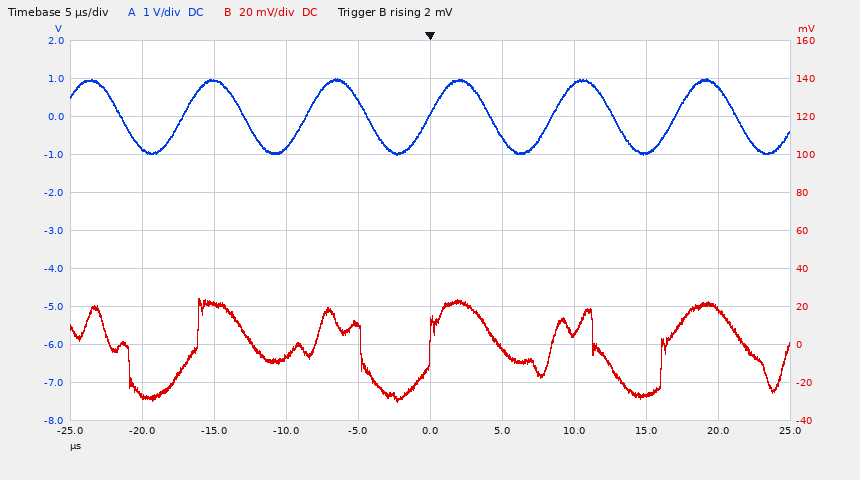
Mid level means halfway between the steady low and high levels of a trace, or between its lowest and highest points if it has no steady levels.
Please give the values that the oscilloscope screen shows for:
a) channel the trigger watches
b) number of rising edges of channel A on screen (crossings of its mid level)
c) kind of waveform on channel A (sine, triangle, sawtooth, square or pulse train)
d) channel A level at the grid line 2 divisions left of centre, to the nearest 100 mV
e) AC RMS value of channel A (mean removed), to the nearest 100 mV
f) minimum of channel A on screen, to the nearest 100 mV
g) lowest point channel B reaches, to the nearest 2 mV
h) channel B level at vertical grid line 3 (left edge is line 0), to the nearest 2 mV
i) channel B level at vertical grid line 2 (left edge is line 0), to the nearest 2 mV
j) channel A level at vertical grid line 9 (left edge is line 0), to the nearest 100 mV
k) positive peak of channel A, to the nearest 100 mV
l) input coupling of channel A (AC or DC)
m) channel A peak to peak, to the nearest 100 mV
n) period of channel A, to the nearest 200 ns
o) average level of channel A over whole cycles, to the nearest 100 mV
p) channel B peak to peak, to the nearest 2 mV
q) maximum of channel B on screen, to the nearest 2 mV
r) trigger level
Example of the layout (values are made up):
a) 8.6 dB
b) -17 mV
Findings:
a) channel B
b) 5
c) sine
d) -800 mV
e) 700 mV
f) -1.0 V
g) -30 mV
h) -6 mV
i) 22 mV
j) 800 mV
k) 1.0 V
l) DC
m) 2.0 V
n) 8.6 µs
o) 0.0 V
p) 54 mV
q) 24 mV
r) 2 mV
